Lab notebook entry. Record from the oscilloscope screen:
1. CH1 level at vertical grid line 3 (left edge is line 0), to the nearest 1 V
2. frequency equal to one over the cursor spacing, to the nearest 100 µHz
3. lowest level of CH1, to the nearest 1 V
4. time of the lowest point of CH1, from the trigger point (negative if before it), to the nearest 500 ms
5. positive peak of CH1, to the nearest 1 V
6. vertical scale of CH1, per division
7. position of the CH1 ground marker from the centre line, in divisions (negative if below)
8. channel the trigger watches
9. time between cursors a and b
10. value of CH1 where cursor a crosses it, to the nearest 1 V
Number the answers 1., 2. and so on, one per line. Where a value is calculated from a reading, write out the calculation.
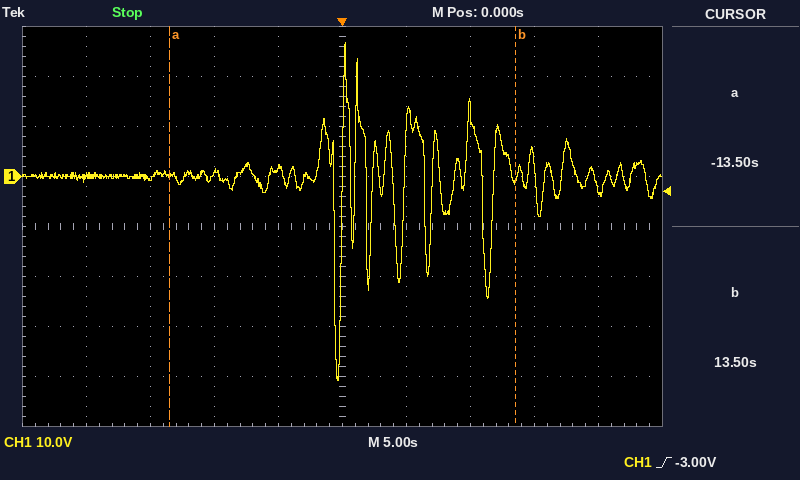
1. 1 V
2. 1 / 27.0 s ≈ 37.0 mHz
3. -41 V
4. -500 ms
5. 27 V
6. 10 V
7. +1.0 div
8. CH1
9. 13.5 s − (-13.5 s) = 27.0 s
10. 0 V
